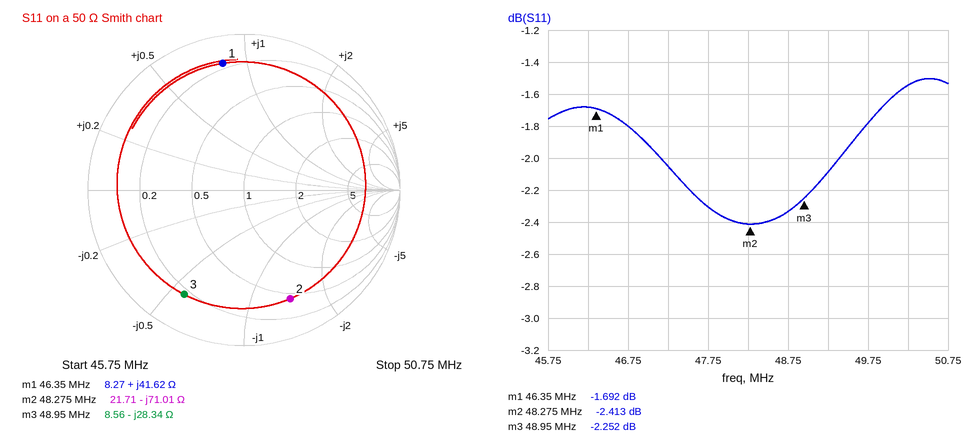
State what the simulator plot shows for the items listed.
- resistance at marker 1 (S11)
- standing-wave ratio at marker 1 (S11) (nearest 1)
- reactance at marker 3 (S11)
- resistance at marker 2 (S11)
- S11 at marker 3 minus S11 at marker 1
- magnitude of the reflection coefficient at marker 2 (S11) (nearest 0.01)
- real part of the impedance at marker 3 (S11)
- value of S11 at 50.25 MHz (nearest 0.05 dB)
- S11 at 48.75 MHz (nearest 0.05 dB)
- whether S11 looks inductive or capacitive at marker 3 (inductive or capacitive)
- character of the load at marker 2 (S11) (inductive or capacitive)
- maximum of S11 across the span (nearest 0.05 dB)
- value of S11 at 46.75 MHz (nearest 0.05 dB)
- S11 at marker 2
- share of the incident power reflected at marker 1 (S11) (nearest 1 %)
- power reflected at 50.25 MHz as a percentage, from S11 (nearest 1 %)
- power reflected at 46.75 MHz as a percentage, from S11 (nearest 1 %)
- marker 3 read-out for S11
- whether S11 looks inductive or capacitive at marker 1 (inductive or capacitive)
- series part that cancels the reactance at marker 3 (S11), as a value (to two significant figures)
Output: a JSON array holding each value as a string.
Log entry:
["8.27 Ω", "10", "-28.34 Ω", "21.71 Ω", "-0.560 dB", "0.76", "8.56 Ω", "-1.55 dB", "-2.35 dB", "capacitive", "capacitive", "-1.50 dB", "-1.80 dB", "-2.413 dB", "68 %", "70 %", "66 %", "-2.252 dB", "inductive", "92 nH"]
